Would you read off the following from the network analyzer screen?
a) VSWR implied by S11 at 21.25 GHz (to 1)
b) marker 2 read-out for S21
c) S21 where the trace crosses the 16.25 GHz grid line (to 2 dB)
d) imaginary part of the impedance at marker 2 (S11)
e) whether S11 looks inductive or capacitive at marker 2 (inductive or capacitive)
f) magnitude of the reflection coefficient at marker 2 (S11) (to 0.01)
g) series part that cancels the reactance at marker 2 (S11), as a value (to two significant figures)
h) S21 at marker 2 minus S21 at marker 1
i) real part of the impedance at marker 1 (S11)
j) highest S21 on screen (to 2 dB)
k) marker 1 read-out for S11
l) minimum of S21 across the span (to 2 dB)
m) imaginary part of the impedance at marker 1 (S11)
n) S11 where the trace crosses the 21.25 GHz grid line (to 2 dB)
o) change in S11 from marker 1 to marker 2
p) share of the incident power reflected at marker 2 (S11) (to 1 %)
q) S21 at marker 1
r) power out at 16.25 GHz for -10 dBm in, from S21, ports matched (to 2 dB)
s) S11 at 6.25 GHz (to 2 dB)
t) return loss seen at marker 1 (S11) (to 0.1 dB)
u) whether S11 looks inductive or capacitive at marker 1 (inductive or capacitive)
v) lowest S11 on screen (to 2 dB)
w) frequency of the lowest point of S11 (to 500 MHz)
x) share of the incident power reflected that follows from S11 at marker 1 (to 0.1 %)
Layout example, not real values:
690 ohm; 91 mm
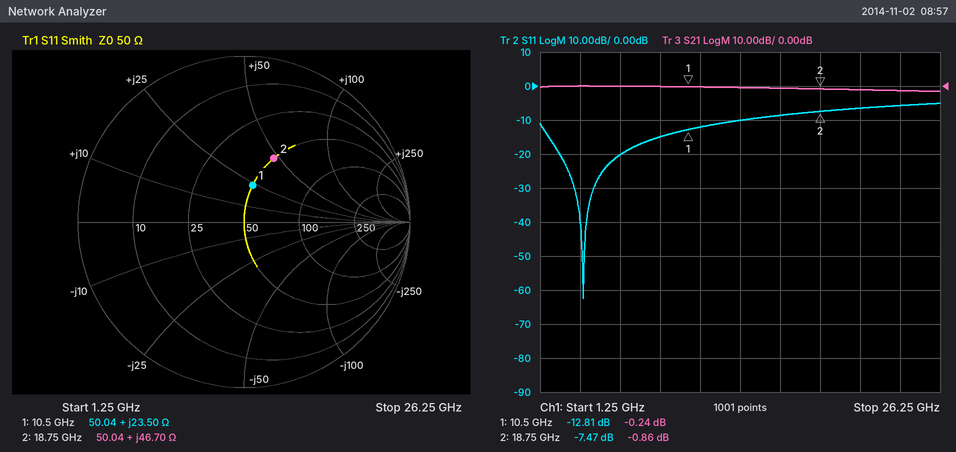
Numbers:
3; -0.86 dB; 0 dB; +46.70 Ω; inductive; 0.42; 180 fF; -0.62 dB; 50.04 Ω; 0 dB; -12.81 dB; -2 dB; +23.50 Ω; -6 dB; 5.34 dB; 18 %; -0.24 dB; -10 dBm; -20 dB; 12.8 dB; inductive; -62 dB; 4.0 GHz; 5.2 %
